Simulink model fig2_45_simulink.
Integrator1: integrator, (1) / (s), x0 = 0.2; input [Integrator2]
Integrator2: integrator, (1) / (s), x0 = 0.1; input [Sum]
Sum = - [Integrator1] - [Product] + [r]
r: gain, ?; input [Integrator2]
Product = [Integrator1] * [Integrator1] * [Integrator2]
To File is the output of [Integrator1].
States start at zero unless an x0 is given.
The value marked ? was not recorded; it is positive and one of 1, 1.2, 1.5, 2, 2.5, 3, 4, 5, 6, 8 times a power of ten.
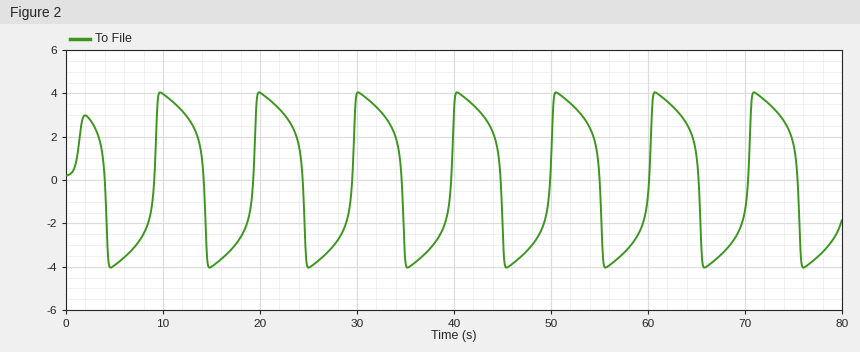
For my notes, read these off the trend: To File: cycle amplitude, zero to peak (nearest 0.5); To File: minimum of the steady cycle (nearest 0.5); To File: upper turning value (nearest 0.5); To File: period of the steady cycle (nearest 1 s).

4.0
-4.0
4.0
10 s
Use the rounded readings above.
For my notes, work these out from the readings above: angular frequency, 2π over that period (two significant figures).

0.63 rad/s
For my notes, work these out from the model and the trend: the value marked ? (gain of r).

4
